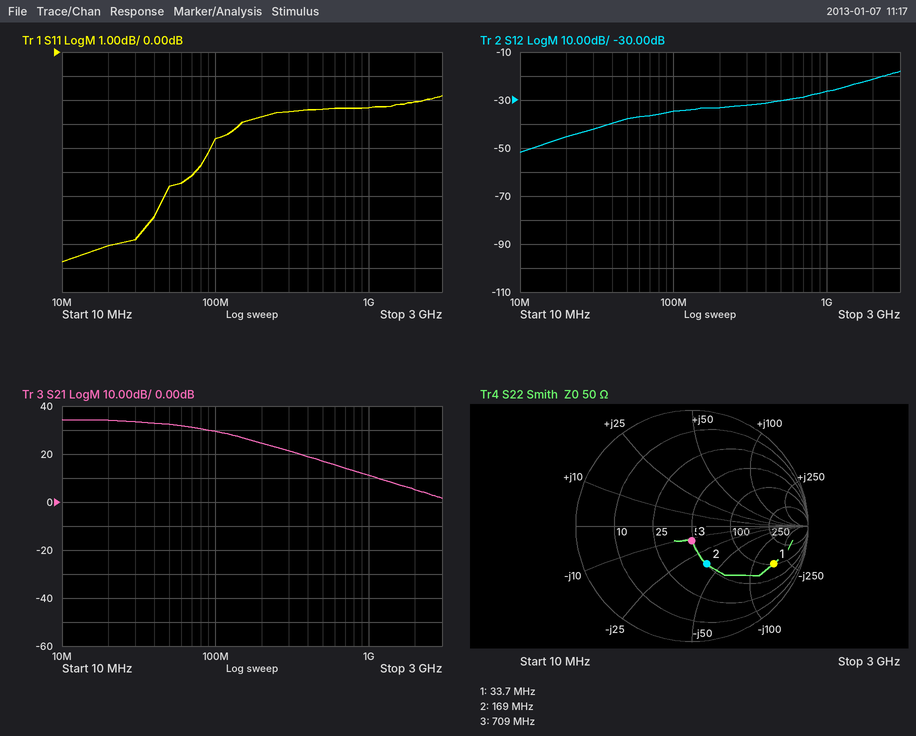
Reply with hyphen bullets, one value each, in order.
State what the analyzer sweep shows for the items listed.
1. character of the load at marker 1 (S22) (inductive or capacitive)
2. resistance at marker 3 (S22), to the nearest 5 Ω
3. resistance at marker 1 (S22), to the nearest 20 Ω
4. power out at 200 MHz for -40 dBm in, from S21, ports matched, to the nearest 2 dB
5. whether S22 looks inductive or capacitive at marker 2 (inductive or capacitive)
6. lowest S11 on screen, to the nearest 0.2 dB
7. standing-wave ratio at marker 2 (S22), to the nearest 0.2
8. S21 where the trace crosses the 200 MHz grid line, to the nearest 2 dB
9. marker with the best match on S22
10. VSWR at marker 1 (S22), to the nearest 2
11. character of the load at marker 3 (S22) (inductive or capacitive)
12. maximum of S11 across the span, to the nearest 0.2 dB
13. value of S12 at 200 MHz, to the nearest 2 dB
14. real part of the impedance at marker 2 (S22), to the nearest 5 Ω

- capacitive
- 50 Ω
- 100 Ω
- -16 dBm
- capacitive
- -8.8 dB
- 2.0
- 24 dB
- marker 3
- 8
- capacitive
- -1.8 dB
- -34 dB
- 50 Ω
